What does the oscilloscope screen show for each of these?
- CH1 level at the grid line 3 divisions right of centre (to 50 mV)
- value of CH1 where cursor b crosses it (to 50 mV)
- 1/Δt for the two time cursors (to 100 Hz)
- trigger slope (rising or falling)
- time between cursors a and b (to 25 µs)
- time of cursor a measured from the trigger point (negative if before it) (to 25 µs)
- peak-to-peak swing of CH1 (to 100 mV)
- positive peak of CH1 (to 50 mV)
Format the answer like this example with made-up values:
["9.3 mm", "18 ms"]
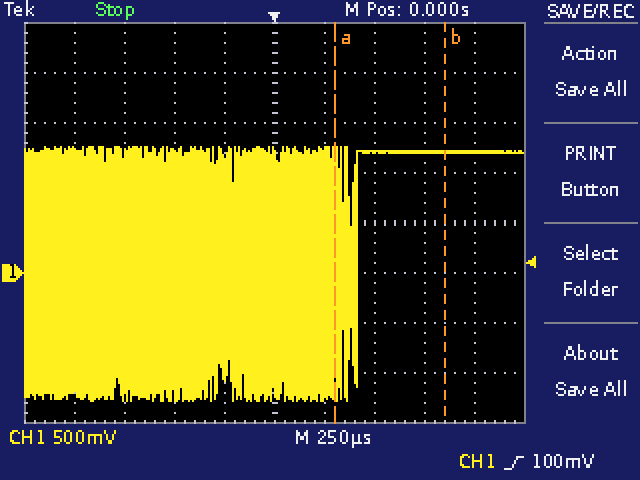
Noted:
["1.20 V", "1.20 V", "1.8 kHz", "rising", "550 µs", "+300 µs", "2.50 V", "1.25 V"]
